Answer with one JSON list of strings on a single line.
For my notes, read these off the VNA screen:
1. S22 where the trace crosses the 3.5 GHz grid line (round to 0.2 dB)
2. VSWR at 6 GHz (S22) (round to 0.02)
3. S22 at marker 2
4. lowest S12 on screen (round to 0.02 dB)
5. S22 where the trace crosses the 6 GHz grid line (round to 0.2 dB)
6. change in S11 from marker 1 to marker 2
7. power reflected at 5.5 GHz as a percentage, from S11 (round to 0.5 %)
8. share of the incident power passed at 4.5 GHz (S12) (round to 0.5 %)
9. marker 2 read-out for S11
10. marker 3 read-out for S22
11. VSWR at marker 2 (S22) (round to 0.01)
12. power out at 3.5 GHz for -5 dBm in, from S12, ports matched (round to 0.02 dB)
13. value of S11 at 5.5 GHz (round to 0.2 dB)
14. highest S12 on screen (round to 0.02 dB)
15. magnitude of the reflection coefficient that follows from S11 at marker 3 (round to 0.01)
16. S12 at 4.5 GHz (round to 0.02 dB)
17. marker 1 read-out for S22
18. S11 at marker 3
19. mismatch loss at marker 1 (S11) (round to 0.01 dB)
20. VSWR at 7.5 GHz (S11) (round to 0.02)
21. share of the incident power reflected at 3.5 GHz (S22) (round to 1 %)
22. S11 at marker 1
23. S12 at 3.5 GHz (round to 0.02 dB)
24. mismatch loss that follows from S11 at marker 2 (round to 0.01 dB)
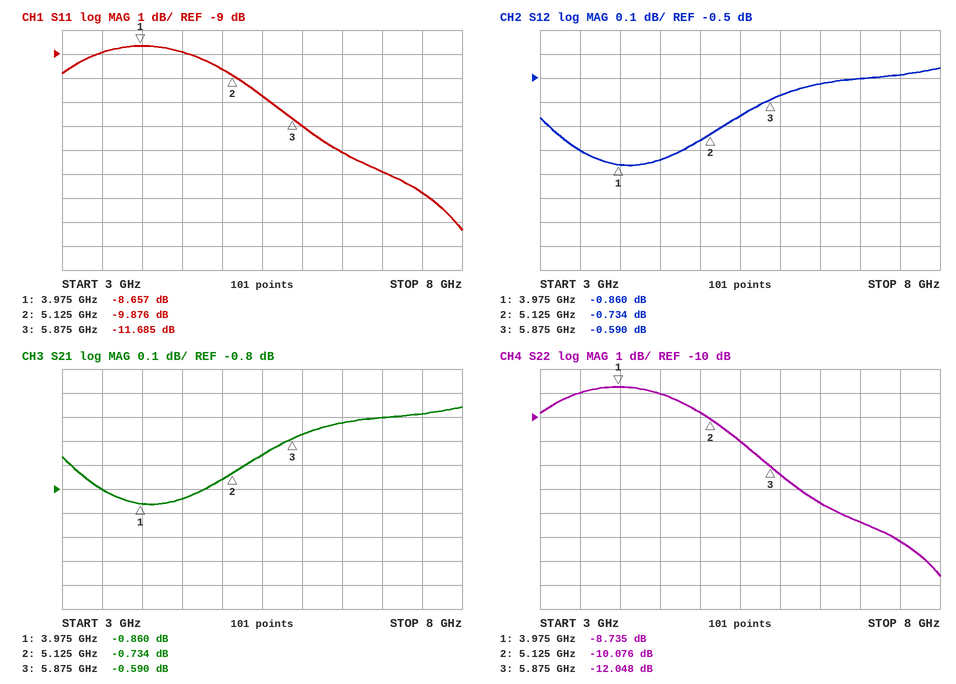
["-9.0 dB", "1.64", "-10.076 dB", "-0.86 dB", "-12.4 dB", "-1.219 dB", "8.5 %", "82.5 %", "-9.876 dB", "-12.048 dB", "1.91", "-5.80 dBm", "-10.8 dB", "-0.46 dB", "0.26", "-0.84 dB", "-8.735 dB", "-11.685 dB", "0.64 dB", "1.44", "13 %", "-8.657 dB", "-0.80 dB", "0.47 dB"]
